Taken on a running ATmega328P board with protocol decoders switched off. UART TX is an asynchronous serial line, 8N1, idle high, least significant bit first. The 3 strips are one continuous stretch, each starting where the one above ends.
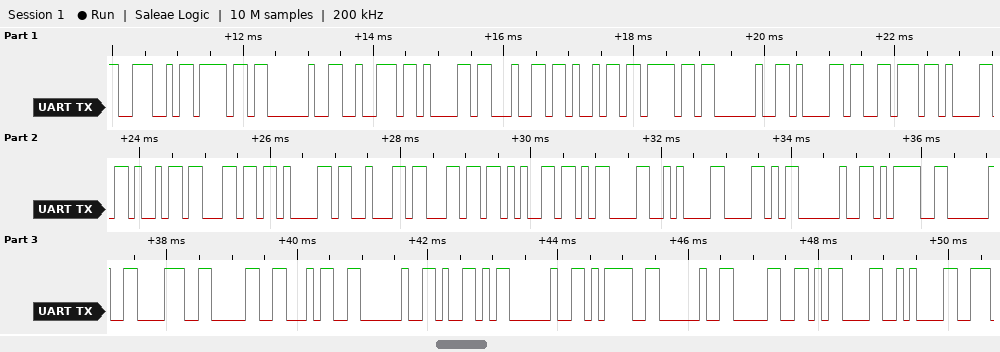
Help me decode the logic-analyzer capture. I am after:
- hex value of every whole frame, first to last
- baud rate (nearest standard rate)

0x4E 0x6F 0x20 0x72 0x61 0x64 0x69 0x6F 0x20 0x61 0x76 0x61 0x69 0x6C 0x61 0x62 0x6C 0x65 0x0D 0x0A 0x58 0x20 0x3D 0x20 0x38 0x30 0x34 0x20 0x59 0x20 0x3D 0x20 0x30 0x0D 0x0A
9600 baud
